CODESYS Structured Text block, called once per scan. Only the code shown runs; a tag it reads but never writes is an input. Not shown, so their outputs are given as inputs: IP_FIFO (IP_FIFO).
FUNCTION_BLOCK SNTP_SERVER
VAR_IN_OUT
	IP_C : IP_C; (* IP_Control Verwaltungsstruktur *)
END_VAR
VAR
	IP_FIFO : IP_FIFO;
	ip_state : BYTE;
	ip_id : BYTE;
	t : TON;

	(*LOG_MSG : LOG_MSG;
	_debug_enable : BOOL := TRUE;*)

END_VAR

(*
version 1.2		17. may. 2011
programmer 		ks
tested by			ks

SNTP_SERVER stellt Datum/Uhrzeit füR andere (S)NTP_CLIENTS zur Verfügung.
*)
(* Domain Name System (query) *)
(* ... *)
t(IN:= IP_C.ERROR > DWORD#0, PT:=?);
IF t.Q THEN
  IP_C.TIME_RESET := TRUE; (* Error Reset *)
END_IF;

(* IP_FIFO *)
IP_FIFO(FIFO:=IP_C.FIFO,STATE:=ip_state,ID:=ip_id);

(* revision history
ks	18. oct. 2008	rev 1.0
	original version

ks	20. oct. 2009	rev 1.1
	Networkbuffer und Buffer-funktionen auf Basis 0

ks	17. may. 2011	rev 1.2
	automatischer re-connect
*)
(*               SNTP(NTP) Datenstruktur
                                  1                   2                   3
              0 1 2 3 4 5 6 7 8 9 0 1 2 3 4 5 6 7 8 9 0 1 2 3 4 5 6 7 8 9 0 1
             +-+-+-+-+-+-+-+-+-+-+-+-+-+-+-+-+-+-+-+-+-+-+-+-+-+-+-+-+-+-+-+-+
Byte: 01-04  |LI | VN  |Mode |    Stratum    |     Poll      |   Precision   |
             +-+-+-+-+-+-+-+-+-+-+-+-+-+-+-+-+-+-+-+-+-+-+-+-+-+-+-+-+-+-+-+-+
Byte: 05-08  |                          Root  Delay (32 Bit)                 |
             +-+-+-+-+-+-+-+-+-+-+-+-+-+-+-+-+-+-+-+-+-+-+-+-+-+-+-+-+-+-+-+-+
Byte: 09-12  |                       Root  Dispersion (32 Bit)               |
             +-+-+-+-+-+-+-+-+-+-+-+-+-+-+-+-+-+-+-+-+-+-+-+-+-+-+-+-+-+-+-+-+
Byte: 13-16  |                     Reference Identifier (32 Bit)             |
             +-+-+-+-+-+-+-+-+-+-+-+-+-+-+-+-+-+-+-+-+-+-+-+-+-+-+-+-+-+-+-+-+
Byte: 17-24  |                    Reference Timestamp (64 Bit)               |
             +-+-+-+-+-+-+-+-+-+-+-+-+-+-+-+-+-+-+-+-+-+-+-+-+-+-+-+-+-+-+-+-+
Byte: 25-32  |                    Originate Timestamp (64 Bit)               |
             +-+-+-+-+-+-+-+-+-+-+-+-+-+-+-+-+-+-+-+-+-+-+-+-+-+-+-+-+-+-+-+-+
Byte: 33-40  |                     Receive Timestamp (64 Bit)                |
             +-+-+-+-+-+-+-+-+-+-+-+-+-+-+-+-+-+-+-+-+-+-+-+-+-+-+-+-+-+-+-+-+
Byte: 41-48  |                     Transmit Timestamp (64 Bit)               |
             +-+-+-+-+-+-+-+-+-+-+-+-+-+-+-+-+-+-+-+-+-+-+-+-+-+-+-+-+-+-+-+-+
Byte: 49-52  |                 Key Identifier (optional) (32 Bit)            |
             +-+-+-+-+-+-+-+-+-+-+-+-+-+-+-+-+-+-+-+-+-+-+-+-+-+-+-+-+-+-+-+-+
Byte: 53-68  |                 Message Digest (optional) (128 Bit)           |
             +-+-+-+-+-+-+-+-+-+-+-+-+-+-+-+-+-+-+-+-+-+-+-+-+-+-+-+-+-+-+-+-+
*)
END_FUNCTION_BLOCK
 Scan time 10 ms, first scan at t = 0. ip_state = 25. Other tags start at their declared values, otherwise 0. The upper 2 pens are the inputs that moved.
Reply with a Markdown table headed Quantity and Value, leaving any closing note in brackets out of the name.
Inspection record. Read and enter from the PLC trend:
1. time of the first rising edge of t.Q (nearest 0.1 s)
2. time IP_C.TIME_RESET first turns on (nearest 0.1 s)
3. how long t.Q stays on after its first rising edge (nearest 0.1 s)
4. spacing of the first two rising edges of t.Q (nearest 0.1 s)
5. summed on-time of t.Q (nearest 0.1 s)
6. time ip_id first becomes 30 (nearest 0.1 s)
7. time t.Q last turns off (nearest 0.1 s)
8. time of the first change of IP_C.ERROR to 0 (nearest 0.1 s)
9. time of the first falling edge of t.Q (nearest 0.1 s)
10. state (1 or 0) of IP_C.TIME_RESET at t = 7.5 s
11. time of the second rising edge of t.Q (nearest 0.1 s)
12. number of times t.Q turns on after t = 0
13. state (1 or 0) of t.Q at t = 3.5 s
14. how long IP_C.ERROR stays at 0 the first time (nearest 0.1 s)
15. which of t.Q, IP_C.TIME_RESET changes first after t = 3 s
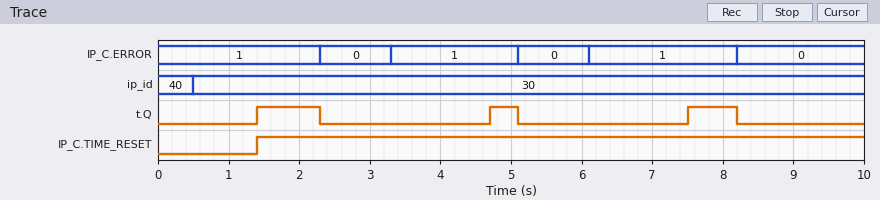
| Quantity | Value |
|---|---|
| time of the first rising edge of t.Q | 1.4 s |
| time IP_C.TIME_RESET first turns on | 1.4 s |
| how long t.Q stays on after its first rising edge | 0.9 s |
| spacing of the first two rising edges of t.Q | 3.3 s |
| summed on-time of t.Q | 2.0 s |
| time ip_id first becomes 30 | 0.5 s |
| time t.Q last turns off | 8.2 s |
| time of the first change of IP_C.ERROR to 0 | 2.3 s |
| time of the first falling edge of t.Q | 2.3 s |
| state (1 or 0) of IP_C.TIME_RESET at t = 7.5 s | 1 |
| time of the second rising edge of t.Q | 4.7 s |
| number of times t.Q turns on after t = 0 | 3 |
| state (1 or 0) of t.Q at t = 3.5 s | 0 |
| how long IP_C.ERROR stays at 0 the first time | 1.0 s |
| which of t.Q, IP_C.TIME_RESET changes first after t = 3 s | t.Q |
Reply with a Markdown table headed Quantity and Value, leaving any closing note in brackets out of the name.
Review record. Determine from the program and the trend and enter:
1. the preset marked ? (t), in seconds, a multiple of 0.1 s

| Quantity | Value |
|---|---|
| the preset marked ? (t), in seconds, a multiple of 0.1 s | 1.4 s |
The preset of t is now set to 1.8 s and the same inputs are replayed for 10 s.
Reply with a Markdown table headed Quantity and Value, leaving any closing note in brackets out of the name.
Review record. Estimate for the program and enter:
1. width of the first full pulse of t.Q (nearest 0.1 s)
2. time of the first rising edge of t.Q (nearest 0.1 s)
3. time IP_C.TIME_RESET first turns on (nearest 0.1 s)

| Quantity | Value |
|---|---|
| width of the first full pulse of t.Q | 0.5 s |
| time of the first rising edge of t.Q | 1.8 s |
| time IP_C.TIME_RESET first turns on | 1.8 s |
